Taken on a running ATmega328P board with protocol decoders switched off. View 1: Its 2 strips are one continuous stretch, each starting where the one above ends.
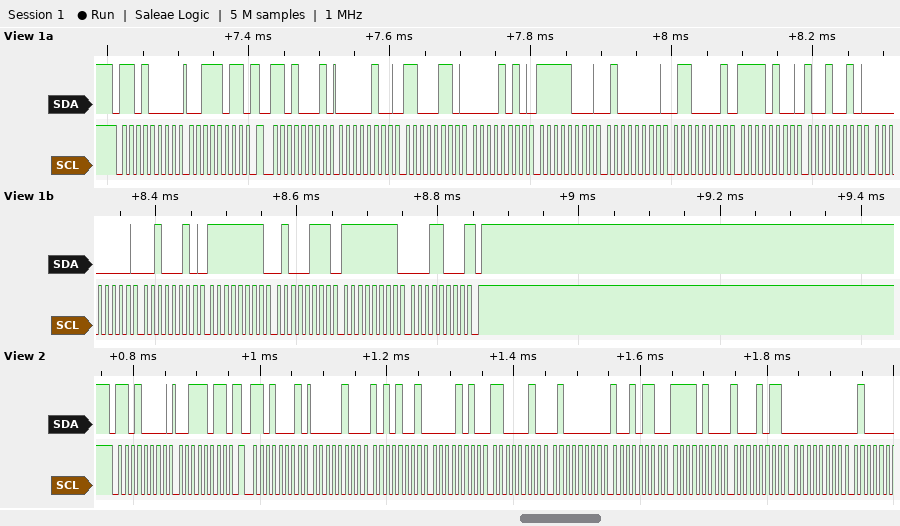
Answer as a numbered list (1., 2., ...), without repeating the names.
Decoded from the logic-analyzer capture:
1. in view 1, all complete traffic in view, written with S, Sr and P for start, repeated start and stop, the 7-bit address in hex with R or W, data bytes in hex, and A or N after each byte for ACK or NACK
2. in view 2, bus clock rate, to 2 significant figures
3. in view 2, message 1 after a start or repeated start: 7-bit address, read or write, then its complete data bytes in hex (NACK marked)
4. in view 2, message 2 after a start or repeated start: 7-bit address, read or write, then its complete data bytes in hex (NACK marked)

1. S 68W A 3B A Sr 68R A 04 A C6 A 0A A F8 A 40 A 61 A F4 A 92 A 00 A 22 A FF A 47 A FF A 18 N P
2. 100 kHz
3. 0x68 write: 3B
4. 0x68 read: 04 A9 0A C2 40 96 F4 8B 00
